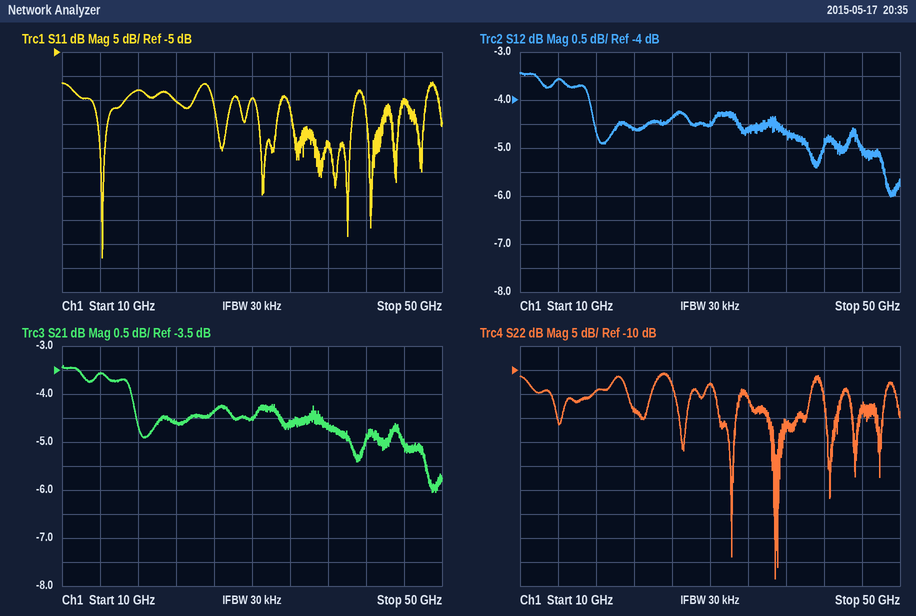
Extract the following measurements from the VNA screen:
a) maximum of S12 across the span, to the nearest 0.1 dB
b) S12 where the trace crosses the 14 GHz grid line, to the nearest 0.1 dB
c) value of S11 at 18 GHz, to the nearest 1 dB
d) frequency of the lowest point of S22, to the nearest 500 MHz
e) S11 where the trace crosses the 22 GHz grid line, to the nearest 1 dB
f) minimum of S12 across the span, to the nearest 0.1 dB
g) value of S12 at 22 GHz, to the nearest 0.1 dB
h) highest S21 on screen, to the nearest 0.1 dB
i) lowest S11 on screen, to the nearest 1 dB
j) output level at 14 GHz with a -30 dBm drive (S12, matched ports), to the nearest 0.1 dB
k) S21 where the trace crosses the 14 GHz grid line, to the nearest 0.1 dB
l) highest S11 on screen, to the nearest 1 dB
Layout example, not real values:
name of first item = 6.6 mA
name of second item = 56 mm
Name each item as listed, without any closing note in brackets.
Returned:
maximum of S12 across the span, to the nearest 0.1 dB = -3.4 dB
S12 where the trace crosses the 14 GHz grid line, to the nearest 0.1 dB = -3.6 dB
value of S11 at 18 GHz, to the nearest 1 dB = -13 dB
frequency of the lowest point of S22, to the nearest 500 MHz = 37.0 GHz
S11 where the trace crosses the 22 GHz grid line, to the nearest 1 dB = -15 dB
minimum of S12 across the span, to the nearest 0.1 dB = -6.0 dB
value of S12 at 22 GHz, to the nearest 0.1 dB = -4.6 dB
highest S21 on screen, to the nearest 0.1 dB = -3.4 dB
lowest S11 on screen, to the nearest 1 dB = -48 dB
output level at 14 GHz with a -30 dBm drive (S12, matched ports), to the nearest 0.1 dB = -33.6 dBm
S21 where the trace crosses the 14 GHz grid line, to the nearest 0.1 dB = -3.6 dB
highest S11 on screen, to the nearest 1 dB = -11 dB
